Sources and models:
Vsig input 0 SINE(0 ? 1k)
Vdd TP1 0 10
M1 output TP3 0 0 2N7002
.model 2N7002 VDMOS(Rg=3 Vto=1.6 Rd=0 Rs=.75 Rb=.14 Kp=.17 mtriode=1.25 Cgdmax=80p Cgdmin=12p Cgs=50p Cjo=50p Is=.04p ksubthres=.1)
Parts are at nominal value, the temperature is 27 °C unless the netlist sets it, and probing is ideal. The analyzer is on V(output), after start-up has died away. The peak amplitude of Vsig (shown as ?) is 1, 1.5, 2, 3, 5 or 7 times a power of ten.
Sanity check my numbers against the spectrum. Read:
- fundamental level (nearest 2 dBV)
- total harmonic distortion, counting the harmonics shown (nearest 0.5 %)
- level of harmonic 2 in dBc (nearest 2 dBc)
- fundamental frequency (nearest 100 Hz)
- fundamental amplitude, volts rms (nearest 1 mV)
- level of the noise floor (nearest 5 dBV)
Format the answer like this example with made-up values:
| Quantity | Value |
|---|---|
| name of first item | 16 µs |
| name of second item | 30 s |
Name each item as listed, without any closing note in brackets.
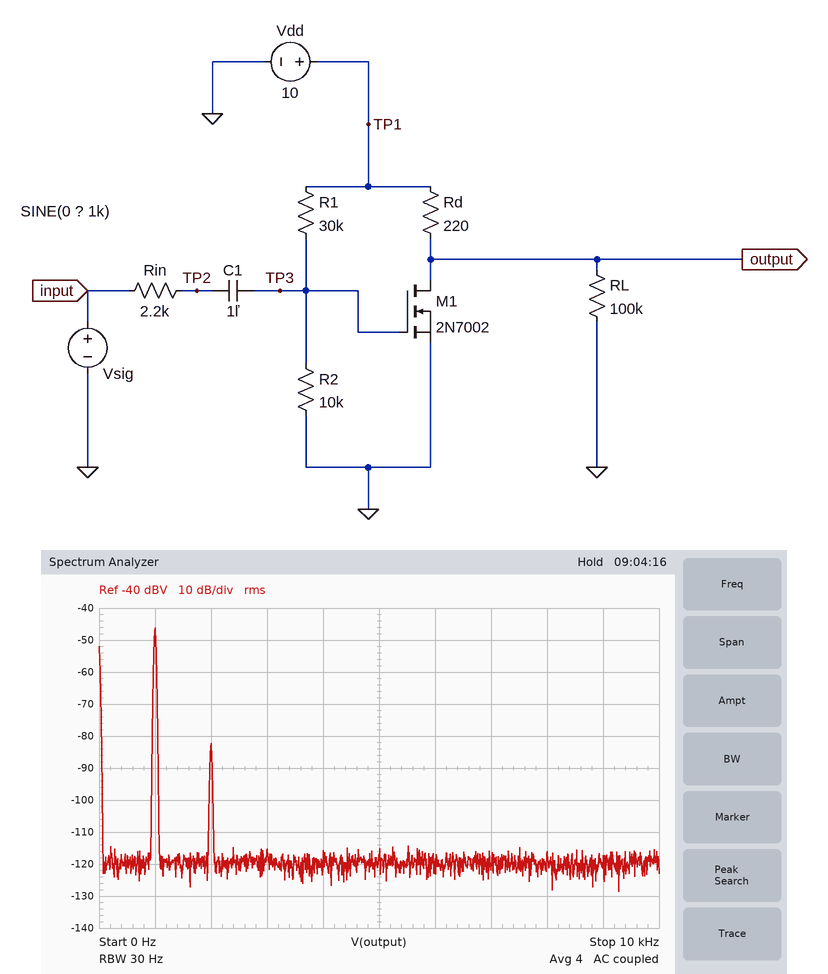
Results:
| Quantity | Value |
|---|---|
| fundamental level | -46 dBV |
| total harmonic distortion, counting the harmonics shown | 1.5 % |
| level of harmonic 2 in dBc | -36 dBc |
| fundamental frequency | 1.0 kHz |
| fundamental amplitude, volts rms | 5 mV |
| level of the noise floor | -120 dBV |
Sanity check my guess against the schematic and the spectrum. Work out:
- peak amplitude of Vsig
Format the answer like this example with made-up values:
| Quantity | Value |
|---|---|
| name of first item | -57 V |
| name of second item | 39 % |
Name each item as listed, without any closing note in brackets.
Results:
| Quantity | Value |
|---|---|
| peak amplitude of Vsig | 15 mV |
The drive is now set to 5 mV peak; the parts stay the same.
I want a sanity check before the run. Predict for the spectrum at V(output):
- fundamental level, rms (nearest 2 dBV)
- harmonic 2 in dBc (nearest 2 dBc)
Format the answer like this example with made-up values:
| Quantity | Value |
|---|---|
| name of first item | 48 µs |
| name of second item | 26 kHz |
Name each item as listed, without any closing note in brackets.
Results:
| Quantity | Value |
|---|---|
| fundamental level, rms | -56 dBV |
| harmonic 2 in dBc | -46 dBc |
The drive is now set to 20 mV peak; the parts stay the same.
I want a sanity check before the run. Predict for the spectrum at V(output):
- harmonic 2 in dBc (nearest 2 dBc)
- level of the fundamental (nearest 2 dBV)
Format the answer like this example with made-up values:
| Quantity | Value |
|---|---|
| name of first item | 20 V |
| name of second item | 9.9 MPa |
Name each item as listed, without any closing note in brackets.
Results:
| Quantity | Value |
|---|---|
| harmonic 2 in dBc | -34 dBc |
| level of the fundamental | -44 dBV |
